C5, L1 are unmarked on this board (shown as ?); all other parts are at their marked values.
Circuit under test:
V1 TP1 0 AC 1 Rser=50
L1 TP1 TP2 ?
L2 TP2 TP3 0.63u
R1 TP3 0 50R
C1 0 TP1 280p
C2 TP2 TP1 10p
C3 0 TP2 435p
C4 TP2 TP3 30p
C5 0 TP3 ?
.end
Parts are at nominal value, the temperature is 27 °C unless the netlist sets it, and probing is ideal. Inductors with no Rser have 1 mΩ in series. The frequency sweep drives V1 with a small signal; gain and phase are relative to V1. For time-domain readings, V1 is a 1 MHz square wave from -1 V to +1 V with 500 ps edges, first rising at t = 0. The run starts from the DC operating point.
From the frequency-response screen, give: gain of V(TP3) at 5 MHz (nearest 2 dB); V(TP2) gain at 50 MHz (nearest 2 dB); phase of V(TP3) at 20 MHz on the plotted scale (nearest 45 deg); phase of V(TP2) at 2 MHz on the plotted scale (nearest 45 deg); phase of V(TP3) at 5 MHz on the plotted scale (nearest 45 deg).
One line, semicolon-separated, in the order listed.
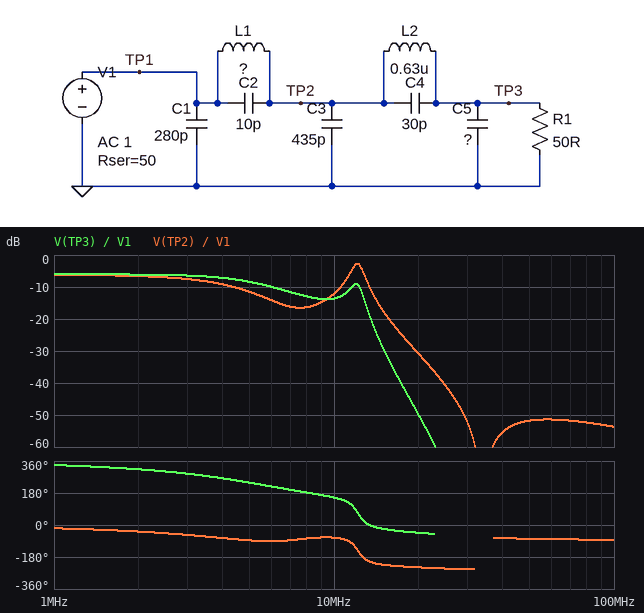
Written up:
-8 dB; -52 dB; -45 deg; -45 deg; 225 deg
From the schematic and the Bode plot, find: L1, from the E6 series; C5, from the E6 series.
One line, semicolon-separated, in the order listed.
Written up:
2.2 µH; 680 pF
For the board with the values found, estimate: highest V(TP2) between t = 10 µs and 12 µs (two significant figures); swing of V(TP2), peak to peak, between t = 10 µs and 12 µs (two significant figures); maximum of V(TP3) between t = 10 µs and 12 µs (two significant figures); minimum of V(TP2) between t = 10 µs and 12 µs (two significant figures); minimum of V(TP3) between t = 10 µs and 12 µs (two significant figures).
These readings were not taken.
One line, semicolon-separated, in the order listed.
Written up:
590 mV; 1.2 V; 570 mV; -590 mV; -570 mV
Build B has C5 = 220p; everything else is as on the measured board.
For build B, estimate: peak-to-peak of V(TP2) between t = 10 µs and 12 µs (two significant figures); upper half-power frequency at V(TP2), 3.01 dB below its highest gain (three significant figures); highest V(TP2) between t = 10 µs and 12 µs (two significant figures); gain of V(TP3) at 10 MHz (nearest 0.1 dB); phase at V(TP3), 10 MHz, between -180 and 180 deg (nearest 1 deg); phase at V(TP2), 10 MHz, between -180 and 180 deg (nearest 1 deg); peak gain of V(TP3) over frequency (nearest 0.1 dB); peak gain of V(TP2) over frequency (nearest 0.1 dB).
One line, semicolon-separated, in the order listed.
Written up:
1.1 V; 6.82 MHz; 530 mV; -12.2 dB; 160 deg; -135 deg; -6.0 dB; -6.0 dB
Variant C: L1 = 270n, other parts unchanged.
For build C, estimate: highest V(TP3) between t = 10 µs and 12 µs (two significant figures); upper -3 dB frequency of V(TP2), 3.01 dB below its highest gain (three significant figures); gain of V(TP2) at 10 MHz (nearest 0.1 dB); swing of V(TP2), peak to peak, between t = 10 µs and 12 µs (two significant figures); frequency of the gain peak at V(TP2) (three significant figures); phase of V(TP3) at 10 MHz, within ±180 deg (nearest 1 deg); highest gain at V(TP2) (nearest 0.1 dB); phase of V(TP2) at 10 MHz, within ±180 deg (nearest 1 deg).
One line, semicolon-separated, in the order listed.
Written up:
540 mV; 24.2 MHz; -5.3 dB; 1.2 V; 21.8 MHz; -159 deg; -1.6 dB; -25 deg
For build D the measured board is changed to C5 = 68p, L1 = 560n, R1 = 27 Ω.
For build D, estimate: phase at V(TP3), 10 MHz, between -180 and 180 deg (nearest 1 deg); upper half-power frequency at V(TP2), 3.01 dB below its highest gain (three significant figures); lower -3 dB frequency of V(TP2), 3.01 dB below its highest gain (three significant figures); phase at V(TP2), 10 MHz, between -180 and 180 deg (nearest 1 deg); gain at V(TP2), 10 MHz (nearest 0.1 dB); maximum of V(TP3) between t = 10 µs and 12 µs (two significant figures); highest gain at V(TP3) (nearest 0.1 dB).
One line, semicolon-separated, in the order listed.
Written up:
-123 deg; 17.5 MHz; 10.9 MHz; -60 deg; -4.7 dB; 470 mV; -8.7 dB
